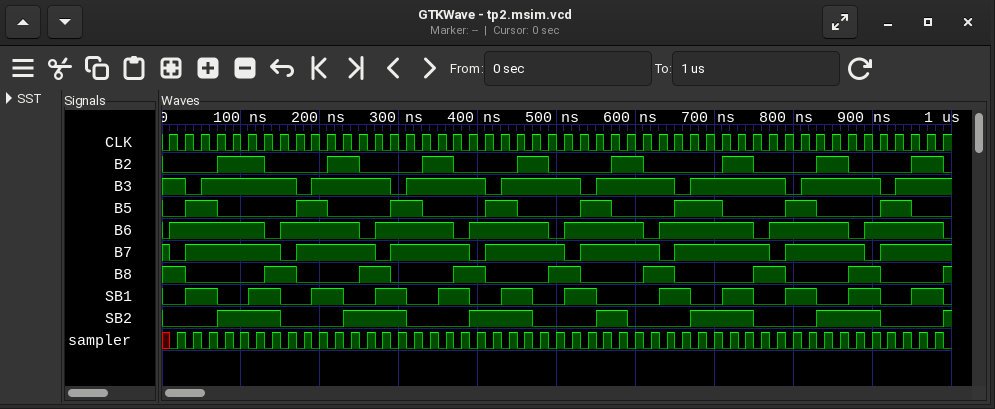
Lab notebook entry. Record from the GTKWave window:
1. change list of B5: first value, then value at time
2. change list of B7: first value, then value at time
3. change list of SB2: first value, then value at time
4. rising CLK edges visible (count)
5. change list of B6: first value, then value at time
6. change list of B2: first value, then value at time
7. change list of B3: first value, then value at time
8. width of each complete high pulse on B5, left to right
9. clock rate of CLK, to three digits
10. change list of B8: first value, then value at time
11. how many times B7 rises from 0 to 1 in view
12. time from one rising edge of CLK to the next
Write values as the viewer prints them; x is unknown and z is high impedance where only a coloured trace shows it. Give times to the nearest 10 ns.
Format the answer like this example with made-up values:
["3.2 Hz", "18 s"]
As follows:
["0, 1 at 30 ns, 0 at 70 ns, 1 at 170 ns, 0 at 210 ns, 1 at 290 ns, 0 at 330 ns, 1 at 410 ns, 0 at 450 ns, 1 at 530 ns, 0 at 570 ns, 1 at 650 ns, 0 at 710 ns, 1 at 790 ns, 0 at 830 ns, 1 at 910 ns, 0 at 950 ns", "1, 0 at 10 ns, 1 at 30 ns, 0 at 150 ns, 1 at 170 ns, 0 at 270 ns, 1 at 290 ns, 0 at 390 ns, 1 at 410 ns, 0 at 510 ns, 1 at 530 ns, 0 at 630 ns, 1 at 650 ns, 0 at 770 ns, 1 at 790 ns, 0 at 890 ns, 1 at 910 ns", "0, 1 at 70 ns, 0 at 150 ns, 1 at 230 ns, 0 at 310 ns, 1 at 390 ns, 0 at 470 ns, 1 at 550 ns, 0 at 590 ns, 1 at 670 ns, 0 at 750 ns, 1 at 830 ns, 0 at 910 ns, 1 at 990 ns", "50", "0, 1 at 10 ns, 0 at 130 ns, 1 at 150 ns, 0 at 250 ns, 1 at 270 ns, 0 at 370 ns, 1 at 390 ns, 0 at 490 ns, 1 at 510 ns, 0 at 610 ns, 1 at 630 ns, 0 at 750 ns, 1 at 770 ns, 0 at 870 ns, 1 at 890 ns, 0 at 990 ns", "0, 1 at 70 ns, 0 at 130 ns, 1 at 210 ns, 0 at 250 ns, 1 at 330 ns, 0 at 370 ns, 1 at 450 ns, 0 at 490 ns, 1 at 570 ns, 0 at 610 ns, 1 at 710 ns, 0 at 750 ns, 1 at 830 ns, 0 at 870 ns, 1 at 950 ns, 0 at 990 ns", "1, 0 at 30 ns, 1 at 50 ns, 0 at 170 ns, 1 at 190 ns, 0 at 290 ns, 1 at 310 ns, 0 at 410 ns, 1 at 430 ns, 0 at 530 ns, 1 at 550 ns, 0 at 650 ns, 1 at 670 ns, 0 at 790 ns, 1 at 810 ns, 0 at 910 ns, 1 at 930 ns", "40 ns, 40 ns, 40 ns, 40 ns, 40 ns, 60 ns, 40 ns, 40 ns", "50.0 MHz", "1, 0 at 30 ns, 1 at 130 ns, 0 at 170 ns, 1 at 250 ns, 0 at 290 ns, 1 at 370 ns, 0 at 410 ns, 1 at 490 ns, 0 at 530 ns, 1 at 610 ns, 0 at 650 ns, 1 at 750 ns, 0 at 790 ns, 1 at 870 ns, 0 at 910 ns, 1 at 990 ns", "8", "20 ns"]
